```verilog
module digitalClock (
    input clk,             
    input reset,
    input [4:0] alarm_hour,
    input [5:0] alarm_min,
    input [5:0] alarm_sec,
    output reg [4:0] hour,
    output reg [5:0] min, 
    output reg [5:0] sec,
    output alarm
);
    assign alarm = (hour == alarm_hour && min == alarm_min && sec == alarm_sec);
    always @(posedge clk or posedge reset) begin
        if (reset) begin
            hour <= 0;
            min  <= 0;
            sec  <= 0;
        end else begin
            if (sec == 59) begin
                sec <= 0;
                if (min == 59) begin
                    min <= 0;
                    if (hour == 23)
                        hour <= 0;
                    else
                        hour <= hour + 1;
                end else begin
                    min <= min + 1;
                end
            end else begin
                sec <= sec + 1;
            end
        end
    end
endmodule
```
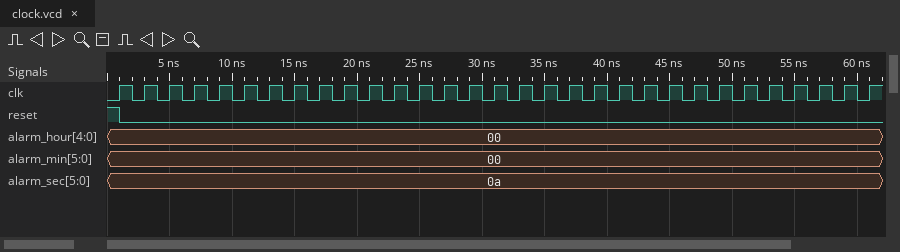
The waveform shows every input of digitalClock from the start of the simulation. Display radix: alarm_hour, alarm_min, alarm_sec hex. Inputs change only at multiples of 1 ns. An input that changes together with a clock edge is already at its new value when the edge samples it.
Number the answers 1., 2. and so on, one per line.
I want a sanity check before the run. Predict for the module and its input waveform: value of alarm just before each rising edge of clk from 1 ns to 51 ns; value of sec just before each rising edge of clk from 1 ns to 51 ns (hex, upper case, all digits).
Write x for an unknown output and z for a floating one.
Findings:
1. 0 0 0 0 0 0 0 0 0 0 1 0 0 0 0 0 0 0 0 0 0 0 0 0 0 0
2. 00, 01, 02, 03, 04, 05, 06, 07, 08, 09, 0A, 0B, 0C, 0D, 0E, 0F, 10, 11, 12, 13, 14, 15, 16, 17, 18, 19
